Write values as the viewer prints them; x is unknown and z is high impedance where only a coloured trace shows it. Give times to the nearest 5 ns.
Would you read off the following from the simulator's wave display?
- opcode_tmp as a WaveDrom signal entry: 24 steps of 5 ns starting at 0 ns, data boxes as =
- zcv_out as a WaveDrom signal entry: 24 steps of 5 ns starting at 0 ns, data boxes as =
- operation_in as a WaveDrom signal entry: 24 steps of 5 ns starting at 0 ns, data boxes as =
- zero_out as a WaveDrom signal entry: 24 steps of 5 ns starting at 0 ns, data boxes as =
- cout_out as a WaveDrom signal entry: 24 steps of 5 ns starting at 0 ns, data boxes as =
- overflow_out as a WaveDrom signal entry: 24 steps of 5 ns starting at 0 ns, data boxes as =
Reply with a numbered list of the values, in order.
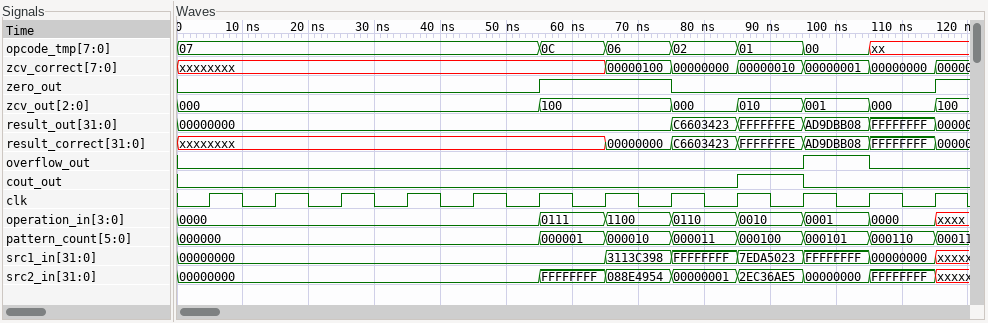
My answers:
1. {name: 'opcode_tmp', wave: '=..........=.=.=.=.=.x..', data: '07 0C 06 02 01 00'}
2. {name: 'zcv_out', wave: '=..........=...=.=.=.=.=', data: '000 100 000 010 001 000 100'}
3. {name: 'operation_in', wave: '=..........=.=.=.=.=.=.x', data: '0000 0111 1100 0110 0010 0001 0000'}
4. {name: 'zero_out', wave: '0..........1...0.......1'}
5. {name: 'cout_out', wave: '0................1.0....'}
6. {name: 'overflow_out', wave: '0..................1.0..'}
